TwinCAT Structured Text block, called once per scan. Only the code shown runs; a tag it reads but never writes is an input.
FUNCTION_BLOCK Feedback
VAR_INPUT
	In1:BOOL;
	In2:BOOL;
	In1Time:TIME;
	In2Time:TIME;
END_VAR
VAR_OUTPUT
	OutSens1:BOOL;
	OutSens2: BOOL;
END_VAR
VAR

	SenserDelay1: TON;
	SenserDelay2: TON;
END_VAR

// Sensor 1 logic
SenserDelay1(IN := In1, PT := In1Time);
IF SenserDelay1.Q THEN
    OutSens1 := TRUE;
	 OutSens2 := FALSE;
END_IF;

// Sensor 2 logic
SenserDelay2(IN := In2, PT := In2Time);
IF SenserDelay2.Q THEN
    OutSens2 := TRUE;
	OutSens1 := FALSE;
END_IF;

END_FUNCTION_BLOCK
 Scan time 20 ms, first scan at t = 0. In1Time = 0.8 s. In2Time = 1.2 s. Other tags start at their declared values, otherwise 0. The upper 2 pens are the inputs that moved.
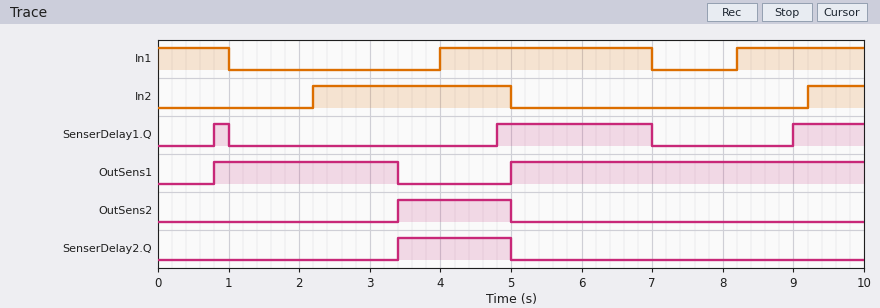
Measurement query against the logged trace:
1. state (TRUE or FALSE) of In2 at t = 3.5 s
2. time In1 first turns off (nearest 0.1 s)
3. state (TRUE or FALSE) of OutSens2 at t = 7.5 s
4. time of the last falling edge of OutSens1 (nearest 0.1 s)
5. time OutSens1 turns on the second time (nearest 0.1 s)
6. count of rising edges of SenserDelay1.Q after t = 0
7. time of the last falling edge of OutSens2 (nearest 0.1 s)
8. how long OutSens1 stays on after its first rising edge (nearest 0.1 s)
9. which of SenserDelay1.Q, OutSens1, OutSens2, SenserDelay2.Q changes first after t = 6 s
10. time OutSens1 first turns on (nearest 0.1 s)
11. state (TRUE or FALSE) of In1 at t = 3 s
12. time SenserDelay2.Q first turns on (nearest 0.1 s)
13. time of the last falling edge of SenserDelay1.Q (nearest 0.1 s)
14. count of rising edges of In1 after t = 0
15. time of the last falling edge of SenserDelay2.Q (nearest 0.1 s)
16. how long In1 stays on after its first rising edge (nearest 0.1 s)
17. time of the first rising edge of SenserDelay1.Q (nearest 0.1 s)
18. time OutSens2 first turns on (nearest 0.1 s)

TRUE
1.0 s
FALSE
3.4 s
5.0 s
3
5.0 s
2.6 s
SenserDelay1.Q
0.8 s
FALSE
3.4 s
7.0 s
2
5.0 s
3.0 s
0.8 s
3.4 s
